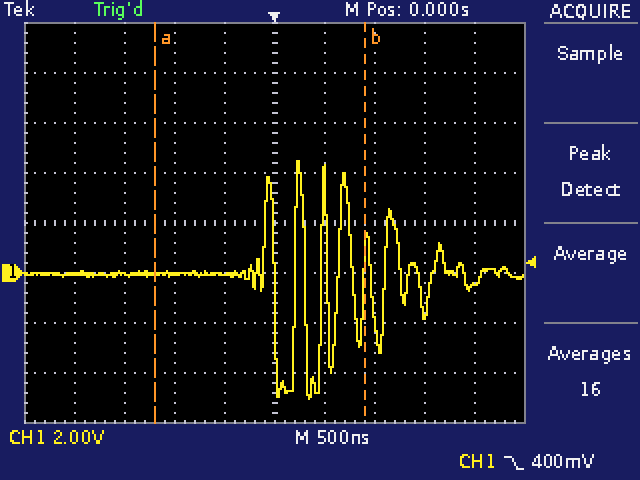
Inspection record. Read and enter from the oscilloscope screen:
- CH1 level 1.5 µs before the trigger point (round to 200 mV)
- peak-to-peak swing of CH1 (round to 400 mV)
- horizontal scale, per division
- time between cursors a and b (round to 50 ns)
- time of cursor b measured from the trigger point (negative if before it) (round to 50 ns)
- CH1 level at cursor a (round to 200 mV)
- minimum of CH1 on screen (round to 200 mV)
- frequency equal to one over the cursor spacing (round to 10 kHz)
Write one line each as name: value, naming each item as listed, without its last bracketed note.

CH1 level 1.5 µs before the trigger point: 0.0 V
peak-to-peak swing of CH1: 9.6 V
horizontal scale, per division: 500 ns
time between cursors a and b: 2.10 µs
time of cursor b measured from the trigger point (negative if before it): +900 ns
CH1 level at cursor a: 0.0 V
minimum of CH1 on screen: -5.0 V
frequency equal to one over the cursor spacing: 480 kHz
